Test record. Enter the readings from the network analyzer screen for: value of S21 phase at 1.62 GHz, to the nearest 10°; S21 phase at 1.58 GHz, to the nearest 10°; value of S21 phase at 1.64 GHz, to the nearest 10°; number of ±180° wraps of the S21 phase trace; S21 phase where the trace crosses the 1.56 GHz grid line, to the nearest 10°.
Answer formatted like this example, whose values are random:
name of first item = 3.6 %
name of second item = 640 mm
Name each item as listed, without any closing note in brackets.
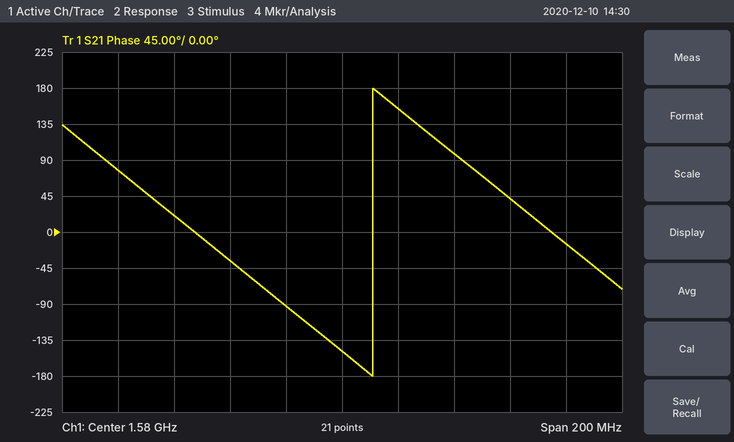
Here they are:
value of S21 phase at 1.62 GHz, to the nearest 10° = 100°
S21 phase at 1.58 GHz, to the nearest 10° = -150°
value of S21 phase at 1.64 GHz, to the nearest 10° = 40°
number of ±180° wraps of the S21 phase trace = 1
S21 phase where the trace crosses the 1.56 GHz grid line, to the nearest 10° = -90°
